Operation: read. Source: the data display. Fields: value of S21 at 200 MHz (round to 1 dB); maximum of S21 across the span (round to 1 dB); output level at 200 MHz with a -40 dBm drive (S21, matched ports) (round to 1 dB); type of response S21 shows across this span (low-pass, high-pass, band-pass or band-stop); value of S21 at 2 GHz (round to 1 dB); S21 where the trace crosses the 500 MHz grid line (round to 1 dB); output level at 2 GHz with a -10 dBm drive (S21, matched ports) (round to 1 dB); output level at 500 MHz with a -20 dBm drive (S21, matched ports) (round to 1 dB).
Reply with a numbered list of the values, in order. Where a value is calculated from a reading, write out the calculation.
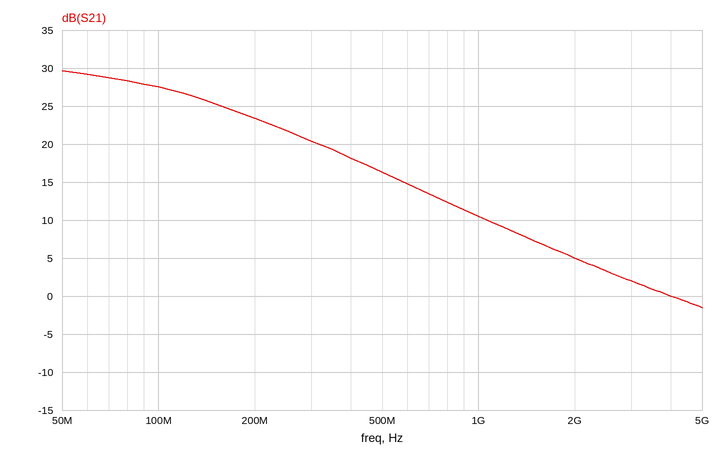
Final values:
1. 23 dB
2. 30 dB
3. -40 dBm + (23 dB) = -17 dBm
4. low-pass
5. 5 dB
6. 16 dB
7. -10 dBm + (5 dB) = -5 dBm
8. -20 dBm + (16 dB) = -4 dBm
